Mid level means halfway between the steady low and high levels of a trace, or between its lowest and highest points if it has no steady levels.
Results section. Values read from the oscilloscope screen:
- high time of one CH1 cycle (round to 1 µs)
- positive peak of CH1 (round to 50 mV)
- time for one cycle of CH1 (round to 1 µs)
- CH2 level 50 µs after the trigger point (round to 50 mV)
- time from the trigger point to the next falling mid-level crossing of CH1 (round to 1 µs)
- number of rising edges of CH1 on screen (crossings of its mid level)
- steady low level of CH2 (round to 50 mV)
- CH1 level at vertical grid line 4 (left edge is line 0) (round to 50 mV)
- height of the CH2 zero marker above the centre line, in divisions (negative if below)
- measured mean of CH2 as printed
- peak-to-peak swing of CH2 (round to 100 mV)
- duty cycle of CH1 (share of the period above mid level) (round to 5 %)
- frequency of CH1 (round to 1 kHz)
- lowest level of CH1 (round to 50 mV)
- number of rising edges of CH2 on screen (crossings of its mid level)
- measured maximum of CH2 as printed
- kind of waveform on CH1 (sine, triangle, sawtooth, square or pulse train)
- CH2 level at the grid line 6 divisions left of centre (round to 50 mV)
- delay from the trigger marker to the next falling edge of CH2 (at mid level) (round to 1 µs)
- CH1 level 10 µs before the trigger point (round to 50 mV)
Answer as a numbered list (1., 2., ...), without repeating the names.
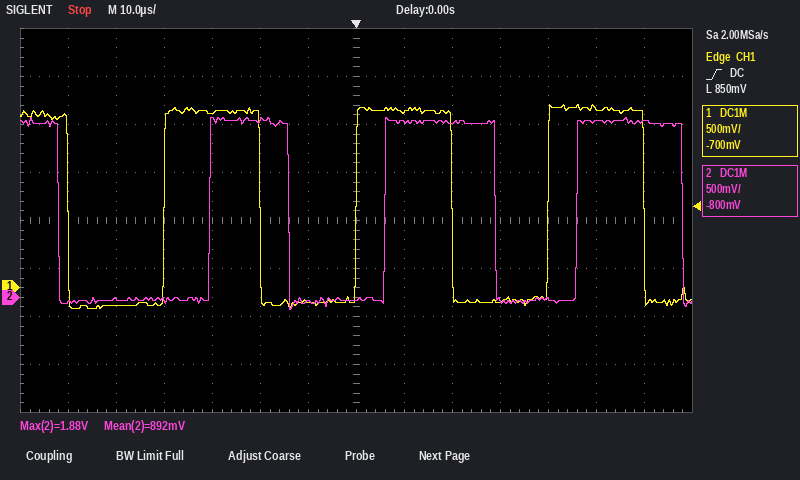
1. 20 µs
2. 1.90 V
3. 40 µs
4. 1.85 V
5. 20 µs
6. 3
7. -50 mV
8. 1.80 V
9. -1.6 div
10. 892 mV
11. 2.00 V
12. 50 %
13. 25 kHz
14. -200 mV
15. 3
16. 1.88 V
17. square
18. -50 mV
19. 29 µs
20. -150 mV
